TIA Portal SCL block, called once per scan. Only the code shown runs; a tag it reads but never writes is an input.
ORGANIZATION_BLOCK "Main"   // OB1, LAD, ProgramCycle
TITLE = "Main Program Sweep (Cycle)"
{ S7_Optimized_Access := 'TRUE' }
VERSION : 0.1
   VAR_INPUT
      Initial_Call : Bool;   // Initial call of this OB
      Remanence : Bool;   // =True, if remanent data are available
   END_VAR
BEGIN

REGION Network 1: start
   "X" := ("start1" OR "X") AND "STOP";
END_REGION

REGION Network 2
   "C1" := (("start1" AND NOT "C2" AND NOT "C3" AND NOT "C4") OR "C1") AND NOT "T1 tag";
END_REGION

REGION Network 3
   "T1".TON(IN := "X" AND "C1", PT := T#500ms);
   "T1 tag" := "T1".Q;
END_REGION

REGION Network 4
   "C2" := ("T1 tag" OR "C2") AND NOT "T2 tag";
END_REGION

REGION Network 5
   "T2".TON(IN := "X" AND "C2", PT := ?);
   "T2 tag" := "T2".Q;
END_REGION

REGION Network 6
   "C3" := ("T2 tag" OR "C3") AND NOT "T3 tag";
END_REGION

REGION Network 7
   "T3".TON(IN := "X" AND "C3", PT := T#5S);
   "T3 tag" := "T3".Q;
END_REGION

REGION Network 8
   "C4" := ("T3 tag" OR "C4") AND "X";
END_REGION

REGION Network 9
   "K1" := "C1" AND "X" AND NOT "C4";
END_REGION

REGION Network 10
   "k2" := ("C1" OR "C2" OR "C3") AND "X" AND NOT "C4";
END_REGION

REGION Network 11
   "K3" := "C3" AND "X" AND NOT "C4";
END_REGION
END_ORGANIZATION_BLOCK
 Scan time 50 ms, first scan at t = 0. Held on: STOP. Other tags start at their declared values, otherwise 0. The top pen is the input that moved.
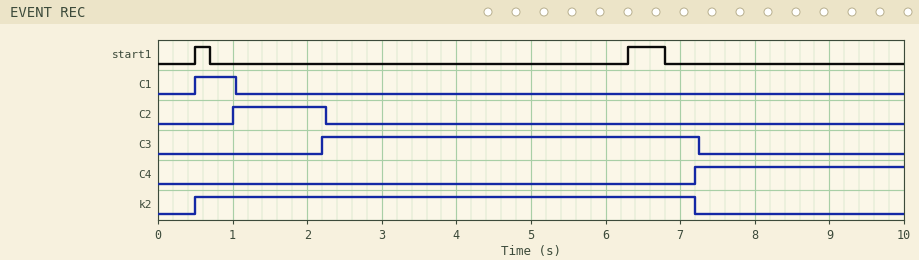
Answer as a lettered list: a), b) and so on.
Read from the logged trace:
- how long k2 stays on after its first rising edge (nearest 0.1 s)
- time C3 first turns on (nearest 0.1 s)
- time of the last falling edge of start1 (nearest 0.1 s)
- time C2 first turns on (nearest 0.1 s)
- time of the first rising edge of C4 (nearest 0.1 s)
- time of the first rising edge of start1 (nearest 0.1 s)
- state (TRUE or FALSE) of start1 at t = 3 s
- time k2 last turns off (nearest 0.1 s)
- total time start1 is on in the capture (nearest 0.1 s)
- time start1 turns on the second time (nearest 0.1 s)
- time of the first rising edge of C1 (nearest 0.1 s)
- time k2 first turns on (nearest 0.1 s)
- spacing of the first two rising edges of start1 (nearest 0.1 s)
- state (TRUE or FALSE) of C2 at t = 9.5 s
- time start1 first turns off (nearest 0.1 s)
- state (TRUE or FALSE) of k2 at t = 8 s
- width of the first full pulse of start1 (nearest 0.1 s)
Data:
a) 6.7 s
b) 2.2 s
c) 6.8 s
d) 1.0 s
e) 7.2 s
f) 0.5 s
g) FALSE
h) 7.2 s
i) 0.7 s
j) 6.3 s
k) 0.5 s
l) 0.5 s
m) 5.8 s
n) FALSE
o) 0.7 s
p) FALSE
q) 0.2 s
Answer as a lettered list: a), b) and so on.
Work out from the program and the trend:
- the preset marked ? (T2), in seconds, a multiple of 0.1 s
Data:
a) 1.2 s
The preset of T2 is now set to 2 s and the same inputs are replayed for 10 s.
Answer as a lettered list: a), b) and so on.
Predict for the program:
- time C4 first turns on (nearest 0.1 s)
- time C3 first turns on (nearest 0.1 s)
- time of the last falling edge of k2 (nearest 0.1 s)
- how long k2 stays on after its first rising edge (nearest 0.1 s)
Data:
a) 8.0 s
b) 3.0 s
c) 8.0 s
d) 7.5 s
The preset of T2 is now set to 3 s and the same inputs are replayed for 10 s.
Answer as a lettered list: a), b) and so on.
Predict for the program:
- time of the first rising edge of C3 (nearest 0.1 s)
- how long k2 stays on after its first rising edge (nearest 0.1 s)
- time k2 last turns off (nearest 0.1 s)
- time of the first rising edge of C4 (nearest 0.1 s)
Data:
a) 4.0 s
b) 8.5 s
c) 9.0 s
d) 9.0 s
